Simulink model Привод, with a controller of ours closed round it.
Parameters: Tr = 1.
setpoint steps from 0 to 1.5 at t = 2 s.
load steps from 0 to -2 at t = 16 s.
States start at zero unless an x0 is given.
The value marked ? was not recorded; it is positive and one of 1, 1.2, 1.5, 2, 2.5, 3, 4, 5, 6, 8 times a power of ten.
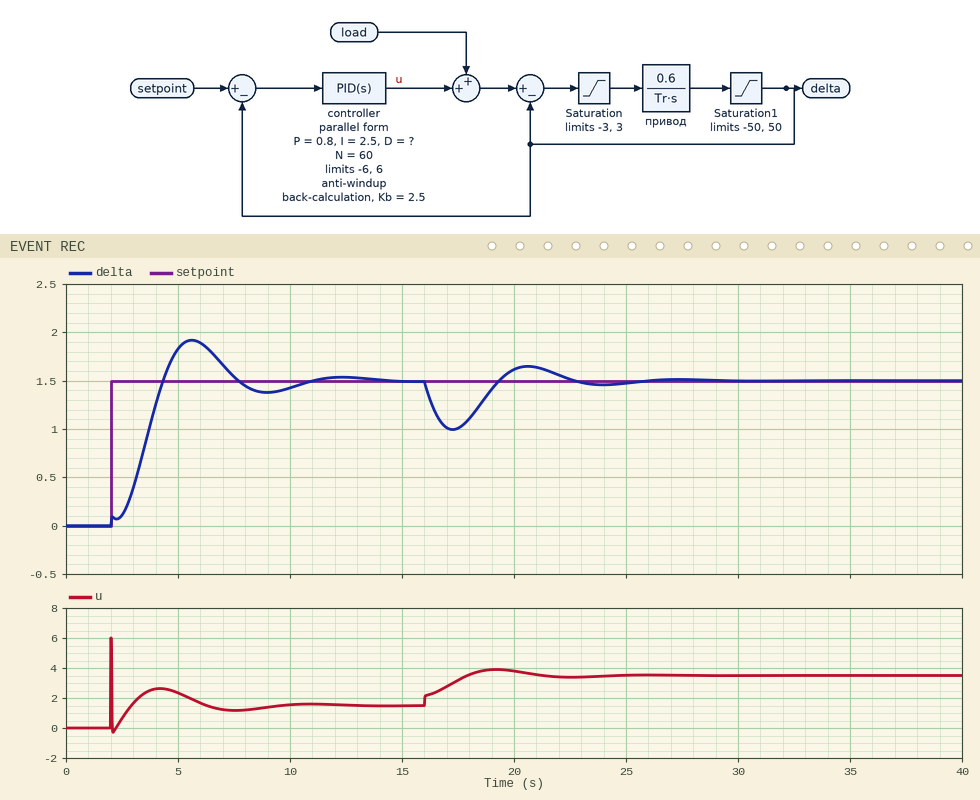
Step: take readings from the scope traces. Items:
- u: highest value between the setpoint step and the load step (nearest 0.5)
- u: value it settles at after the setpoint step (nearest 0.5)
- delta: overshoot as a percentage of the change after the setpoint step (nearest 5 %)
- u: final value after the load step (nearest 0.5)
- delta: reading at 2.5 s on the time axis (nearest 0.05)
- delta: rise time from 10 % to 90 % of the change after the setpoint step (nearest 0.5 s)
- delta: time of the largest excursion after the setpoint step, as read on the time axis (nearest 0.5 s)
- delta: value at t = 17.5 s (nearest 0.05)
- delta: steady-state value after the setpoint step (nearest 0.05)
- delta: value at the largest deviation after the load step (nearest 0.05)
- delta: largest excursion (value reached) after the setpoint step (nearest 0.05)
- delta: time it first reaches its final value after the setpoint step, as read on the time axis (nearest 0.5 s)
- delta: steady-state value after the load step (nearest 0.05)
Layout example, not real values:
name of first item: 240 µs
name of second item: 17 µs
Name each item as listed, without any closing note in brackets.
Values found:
u: highest value between the setpoint step and the load step: 6.0
u: value it settles at after the setpoint step: 1.5
delta: overshoot as a percentage of the change after the setpoint step: 30 %
u: final value after the load step: 3.5
delta: reading at 2.5 s on the time axis: 0.10
delta: rise time from 10 % to 90 % of the change after the setpoint step: 1.5 s
delta: time of the largest excursion after the setpoint step, as read on the time axis: 5.5 s
delta: value at t = 17.5 s: 1.00
delta: steady-state value after the setpoint step: 1.50
delta: value at the largest deviation after the load step: 1.00
delta: largest excursion (value reached) after the setpoint step: 1.90
delta: time it first reaches its final value after the setpoint step, as read on the time axis: 4.5 s
delta: steady-state value after the load step: 1.50
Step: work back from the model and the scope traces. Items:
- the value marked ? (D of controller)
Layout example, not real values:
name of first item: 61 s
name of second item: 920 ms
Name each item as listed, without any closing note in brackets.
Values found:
the value marked ?: 0.8
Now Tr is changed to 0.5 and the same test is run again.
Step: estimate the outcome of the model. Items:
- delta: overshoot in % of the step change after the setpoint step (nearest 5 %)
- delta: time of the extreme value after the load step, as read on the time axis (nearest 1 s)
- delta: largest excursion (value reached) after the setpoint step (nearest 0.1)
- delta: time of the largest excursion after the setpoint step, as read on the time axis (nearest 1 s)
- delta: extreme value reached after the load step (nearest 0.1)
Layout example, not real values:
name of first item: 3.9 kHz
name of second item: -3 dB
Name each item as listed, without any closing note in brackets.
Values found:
delta: overshoot in % of the step change after the setpoint step: 20 %
delta: time of the extreme value after the load step, as read on the time axis: 17 s
delta: largest excursion (value reached) after the setpoint step: 1.8
delta: time of the largest excursion after the setpoint step, as read on the time axis: 5 s
delta: extreme value reached after the load step: 0.9
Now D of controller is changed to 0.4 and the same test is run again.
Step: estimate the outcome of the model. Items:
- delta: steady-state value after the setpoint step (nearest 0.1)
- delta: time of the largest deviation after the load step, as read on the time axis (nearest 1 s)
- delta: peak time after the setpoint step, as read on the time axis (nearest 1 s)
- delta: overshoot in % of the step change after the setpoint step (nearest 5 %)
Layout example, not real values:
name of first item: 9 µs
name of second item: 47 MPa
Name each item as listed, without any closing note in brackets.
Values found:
delta: steady-state value after the setpoint step: 1.5
delta: time of the largest deviation after the load step, as read on the time axis: 17 s
delta: peak time after the setpoint step, as read on the time axis: 5 s
delta: overshoot in % of the step change after the setpoint step: 25 %
